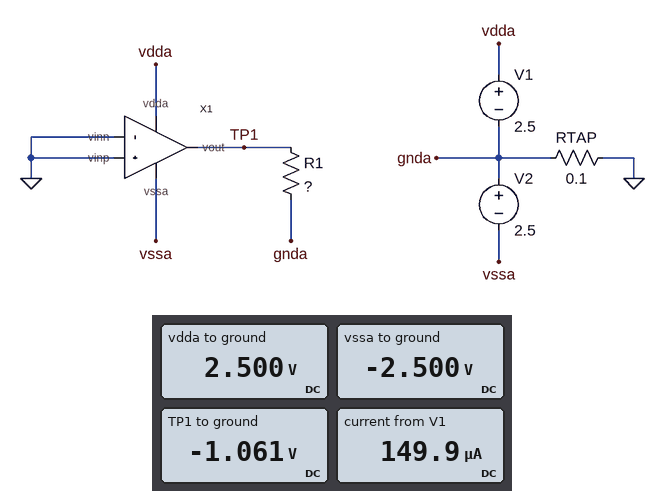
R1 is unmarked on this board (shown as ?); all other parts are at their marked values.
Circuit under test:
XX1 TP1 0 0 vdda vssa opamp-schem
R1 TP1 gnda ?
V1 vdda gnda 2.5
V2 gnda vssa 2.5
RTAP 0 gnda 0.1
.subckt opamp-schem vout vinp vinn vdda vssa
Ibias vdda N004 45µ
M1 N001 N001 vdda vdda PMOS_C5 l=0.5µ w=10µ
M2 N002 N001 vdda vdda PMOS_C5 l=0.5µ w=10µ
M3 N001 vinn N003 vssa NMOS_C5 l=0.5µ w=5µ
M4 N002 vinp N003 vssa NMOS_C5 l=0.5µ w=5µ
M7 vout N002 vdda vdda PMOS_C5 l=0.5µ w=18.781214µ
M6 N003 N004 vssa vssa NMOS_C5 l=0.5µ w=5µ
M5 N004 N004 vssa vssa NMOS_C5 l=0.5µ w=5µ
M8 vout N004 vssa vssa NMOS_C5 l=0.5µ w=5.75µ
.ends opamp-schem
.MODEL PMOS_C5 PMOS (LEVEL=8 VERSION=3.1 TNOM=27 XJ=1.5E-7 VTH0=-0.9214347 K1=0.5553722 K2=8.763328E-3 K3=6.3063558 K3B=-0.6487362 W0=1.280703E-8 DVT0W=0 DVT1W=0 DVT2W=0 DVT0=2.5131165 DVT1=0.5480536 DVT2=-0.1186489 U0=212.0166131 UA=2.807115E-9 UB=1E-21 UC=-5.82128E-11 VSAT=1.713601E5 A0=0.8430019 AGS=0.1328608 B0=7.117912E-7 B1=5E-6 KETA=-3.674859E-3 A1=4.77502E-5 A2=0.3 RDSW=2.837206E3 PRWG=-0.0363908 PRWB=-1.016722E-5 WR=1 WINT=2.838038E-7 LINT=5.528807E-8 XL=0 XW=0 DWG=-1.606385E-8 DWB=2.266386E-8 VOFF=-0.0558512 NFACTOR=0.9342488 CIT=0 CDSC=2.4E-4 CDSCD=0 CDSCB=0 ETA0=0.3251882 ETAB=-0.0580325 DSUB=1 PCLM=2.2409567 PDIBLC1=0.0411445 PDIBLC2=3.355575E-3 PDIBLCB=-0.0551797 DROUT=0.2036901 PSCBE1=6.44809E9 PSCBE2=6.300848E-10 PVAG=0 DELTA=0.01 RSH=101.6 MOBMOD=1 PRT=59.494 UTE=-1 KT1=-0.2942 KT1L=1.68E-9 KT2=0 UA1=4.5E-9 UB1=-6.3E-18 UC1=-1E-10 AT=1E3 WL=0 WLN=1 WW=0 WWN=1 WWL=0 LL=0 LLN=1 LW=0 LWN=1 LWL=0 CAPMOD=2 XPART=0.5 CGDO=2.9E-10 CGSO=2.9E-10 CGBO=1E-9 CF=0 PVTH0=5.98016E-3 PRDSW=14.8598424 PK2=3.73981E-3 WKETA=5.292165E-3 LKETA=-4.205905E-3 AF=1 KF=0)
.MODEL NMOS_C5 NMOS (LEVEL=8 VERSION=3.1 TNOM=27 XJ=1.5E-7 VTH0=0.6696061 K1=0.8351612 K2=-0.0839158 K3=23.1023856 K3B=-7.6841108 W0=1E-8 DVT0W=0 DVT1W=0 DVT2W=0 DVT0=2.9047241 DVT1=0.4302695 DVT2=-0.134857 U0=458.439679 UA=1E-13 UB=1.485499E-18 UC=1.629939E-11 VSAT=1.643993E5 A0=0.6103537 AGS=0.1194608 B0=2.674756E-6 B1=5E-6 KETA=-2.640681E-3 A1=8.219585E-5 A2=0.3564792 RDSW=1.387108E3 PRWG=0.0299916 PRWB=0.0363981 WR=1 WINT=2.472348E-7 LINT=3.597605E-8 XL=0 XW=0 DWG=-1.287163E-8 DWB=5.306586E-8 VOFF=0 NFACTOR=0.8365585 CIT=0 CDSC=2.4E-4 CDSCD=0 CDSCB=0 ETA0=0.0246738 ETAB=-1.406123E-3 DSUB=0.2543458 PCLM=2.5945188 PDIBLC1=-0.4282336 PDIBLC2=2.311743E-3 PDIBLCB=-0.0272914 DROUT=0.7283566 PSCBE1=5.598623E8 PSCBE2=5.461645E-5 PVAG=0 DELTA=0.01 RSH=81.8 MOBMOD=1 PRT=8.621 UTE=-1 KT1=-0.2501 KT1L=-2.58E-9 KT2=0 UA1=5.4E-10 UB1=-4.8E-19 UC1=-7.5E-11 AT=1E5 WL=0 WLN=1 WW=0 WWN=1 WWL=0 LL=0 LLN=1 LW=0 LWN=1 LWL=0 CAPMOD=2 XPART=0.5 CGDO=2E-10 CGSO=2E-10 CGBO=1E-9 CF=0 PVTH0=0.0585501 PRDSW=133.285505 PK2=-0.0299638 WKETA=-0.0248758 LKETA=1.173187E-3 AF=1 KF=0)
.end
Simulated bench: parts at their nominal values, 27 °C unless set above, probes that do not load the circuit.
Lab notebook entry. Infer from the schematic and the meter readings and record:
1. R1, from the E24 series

390 kΩ
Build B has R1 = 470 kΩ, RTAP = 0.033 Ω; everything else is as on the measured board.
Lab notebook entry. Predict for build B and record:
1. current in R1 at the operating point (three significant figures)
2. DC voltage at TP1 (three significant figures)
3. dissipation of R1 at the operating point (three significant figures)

2.32 µA
-1.09 V
2.54 µW
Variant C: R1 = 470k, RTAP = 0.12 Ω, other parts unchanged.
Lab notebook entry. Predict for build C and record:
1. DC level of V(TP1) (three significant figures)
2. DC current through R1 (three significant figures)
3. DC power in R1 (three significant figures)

-1.09 V
2.32 µA
2.54 µW
